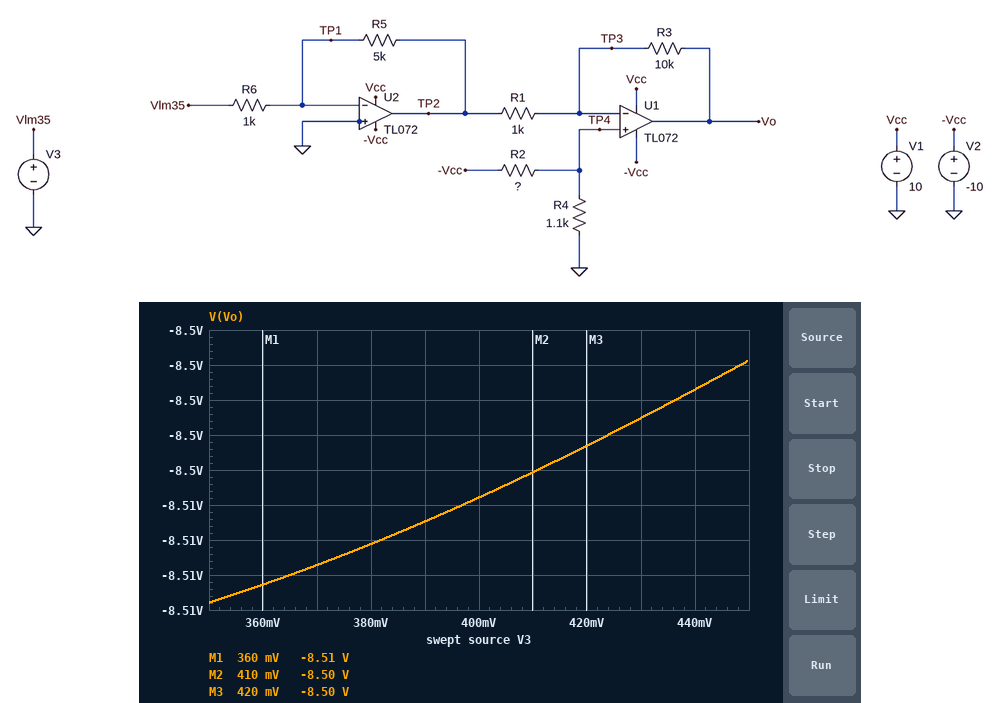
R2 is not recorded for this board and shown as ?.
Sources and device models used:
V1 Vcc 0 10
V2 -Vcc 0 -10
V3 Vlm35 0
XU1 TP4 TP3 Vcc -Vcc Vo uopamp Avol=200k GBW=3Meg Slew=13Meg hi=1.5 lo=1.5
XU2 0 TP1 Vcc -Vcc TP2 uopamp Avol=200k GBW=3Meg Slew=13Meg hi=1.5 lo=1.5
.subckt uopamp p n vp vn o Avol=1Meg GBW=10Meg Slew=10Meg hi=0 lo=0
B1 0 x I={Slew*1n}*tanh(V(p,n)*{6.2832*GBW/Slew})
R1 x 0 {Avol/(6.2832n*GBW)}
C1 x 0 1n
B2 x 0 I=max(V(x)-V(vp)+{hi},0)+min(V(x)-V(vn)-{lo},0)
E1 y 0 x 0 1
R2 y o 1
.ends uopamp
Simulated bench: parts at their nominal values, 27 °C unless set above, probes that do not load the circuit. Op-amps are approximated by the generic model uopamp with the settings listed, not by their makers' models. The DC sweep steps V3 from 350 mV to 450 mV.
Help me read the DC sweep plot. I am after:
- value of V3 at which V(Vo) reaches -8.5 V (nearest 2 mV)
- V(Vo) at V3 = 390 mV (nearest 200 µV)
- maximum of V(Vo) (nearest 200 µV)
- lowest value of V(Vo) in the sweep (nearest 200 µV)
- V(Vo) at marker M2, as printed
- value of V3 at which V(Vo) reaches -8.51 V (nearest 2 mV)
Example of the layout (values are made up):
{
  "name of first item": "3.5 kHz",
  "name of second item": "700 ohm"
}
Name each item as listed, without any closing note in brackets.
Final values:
{
  "value of V3 at which V(Vo) reaches -8.5 V": "424 mV",
  "V(Vo) at V3 = 390 mV": "-8.5054 V",
  "maximum of V(Vo)": "-8.5008 V",
  "lowest value of V(Vo) in the sweep": "-8.5078 V",
  "V(Vo) at marker M2, as printed": "-8.50 V",
  "value of V3 at which V(Vo) reaches -8.51 V": "382 mV"
}
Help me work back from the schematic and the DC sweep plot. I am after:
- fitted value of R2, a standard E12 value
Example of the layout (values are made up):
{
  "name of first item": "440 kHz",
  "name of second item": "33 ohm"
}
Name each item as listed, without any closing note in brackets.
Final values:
{
  "fitted value of R2, a standard E12 value": "2.7 kΩ"
}
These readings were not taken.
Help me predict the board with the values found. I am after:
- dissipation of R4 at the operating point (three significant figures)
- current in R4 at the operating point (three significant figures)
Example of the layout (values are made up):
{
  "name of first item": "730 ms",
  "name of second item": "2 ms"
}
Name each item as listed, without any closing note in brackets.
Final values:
{
  "dissipation of R4 at the operating point": "7.62 mW",
  "current in R4 at the operating point": "2.63 mA"
}
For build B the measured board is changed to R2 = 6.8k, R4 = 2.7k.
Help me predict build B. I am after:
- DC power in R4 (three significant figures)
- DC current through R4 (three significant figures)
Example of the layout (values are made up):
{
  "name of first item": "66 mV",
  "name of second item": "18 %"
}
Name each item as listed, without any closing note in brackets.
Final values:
{
  "DC power in R4": "2.99 mW",
  "DC current through R4": "1.05 mA"
}
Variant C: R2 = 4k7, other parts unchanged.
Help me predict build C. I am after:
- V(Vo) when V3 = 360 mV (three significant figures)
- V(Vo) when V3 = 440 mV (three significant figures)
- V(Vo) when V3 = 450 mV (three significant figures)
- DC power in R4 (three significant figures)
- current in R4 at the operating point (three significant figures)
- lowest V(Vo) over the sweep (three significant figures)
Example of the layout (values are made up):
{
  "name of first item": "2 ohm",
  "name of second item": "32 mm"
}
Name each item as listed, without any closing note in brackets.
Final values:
{
  "V(Vo) when V3 = 360 mV": "-2.86 V",
  "V(Vo) when V3 = 440 mV": "1.14 V",
  "V(Vo) when V3 = 450 mV": "1.64 V",
  "DC power in R4": "3.27 mW",
  "current in R4 at the operating point": "1.72 mA",
  "lowest V(Vo) over the sweep": "-3.36 V"
}
